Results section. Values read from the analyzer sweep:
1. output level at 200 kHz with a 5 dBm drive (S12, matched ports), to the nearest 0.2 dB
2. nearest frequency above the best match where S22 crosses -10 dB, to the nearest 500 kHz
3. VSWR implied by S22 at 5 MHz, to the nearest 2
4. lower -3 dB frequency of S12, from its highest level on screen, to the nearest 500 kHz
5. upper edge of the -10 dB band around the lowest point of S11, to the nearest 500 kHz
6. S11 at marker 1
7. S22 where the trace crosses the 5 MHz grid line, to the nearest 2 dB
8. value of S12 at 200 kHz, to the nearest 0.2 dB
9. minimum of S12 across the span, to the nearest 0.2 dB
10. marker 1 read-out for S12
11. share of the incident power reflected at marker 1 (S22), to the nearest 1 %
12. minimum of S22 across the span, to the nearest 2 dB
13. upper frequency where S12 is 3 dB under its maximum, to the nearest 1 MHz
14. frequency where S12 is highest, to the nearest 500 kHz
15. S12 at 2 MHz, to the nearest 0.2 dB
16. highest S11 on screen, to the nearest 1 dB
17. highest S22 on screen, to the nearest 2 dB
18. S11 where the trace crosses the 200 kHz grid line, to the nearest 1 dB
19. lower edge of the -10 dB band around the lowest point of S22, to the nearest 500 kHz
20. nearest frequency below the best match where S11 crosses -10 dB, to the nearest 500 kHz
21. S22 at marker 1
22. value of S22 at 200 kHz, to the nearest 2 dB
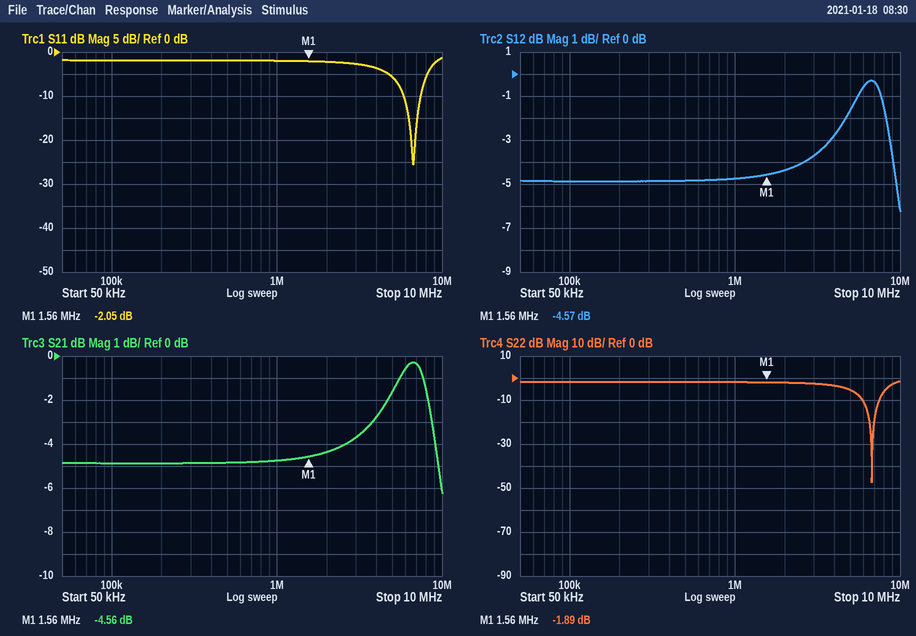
0.2 dBm
7.5 MHz
4
3.5 MHz
7.5 MHz
-2.05 dB
-6 dB
-4.8 dB
-6.2 dB
-4.57 dB
65 %
-48 dB
9 MHz
6.5 MHz
-4.4 dB
-1 dB
-2 dB
-2 dB
6.0 MHz
6.0 MHz
-1.89 dB
-2 dB
